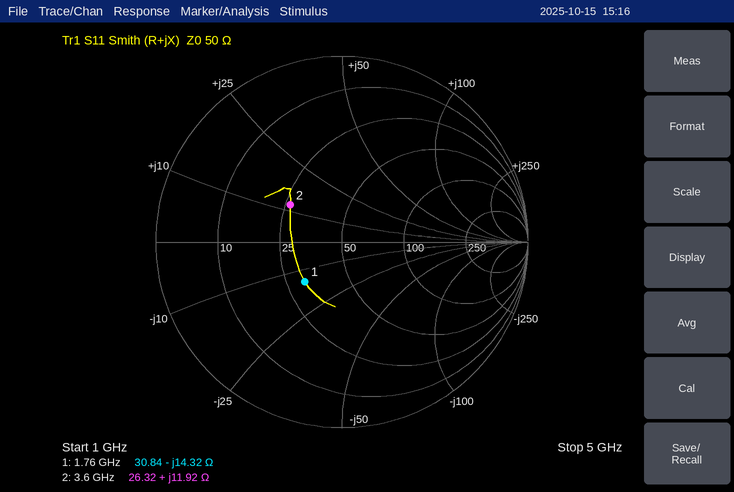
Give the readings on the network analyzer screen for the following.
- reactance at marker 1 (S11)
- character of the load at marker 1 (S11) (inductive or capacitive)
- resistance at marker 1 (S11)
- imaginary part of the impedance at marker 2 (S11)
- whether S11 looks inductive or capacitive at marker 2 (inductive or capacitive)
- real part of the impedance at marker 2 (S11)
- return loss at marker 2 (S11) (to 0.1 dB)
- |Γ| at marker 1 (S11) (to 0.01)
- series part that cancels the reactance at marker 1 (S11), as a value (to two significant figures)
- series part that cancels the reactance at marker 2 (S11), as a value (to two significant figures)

-14.32 Ω
capacitive
30.84 Ω
+11.92 Ω
inductive
26.32 Ω
9.3 dB
0.29
1.3 nH
3.7 pF
